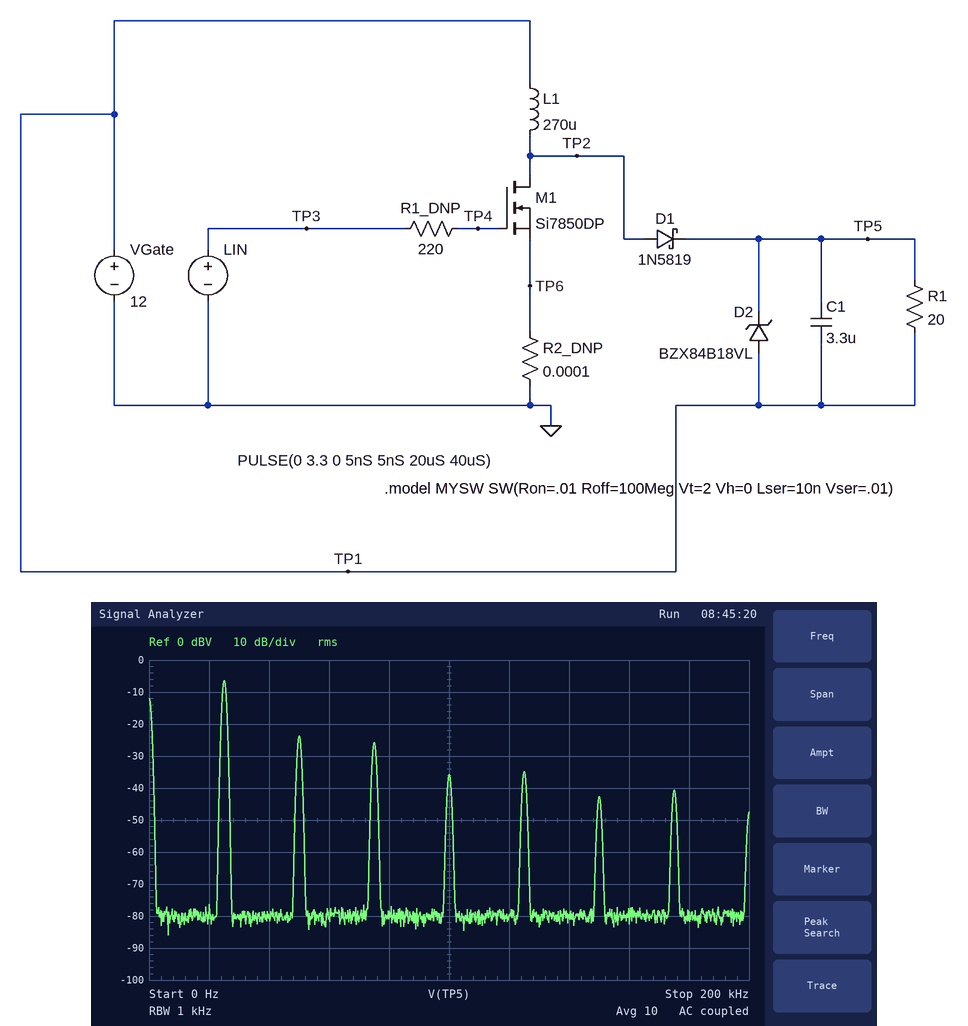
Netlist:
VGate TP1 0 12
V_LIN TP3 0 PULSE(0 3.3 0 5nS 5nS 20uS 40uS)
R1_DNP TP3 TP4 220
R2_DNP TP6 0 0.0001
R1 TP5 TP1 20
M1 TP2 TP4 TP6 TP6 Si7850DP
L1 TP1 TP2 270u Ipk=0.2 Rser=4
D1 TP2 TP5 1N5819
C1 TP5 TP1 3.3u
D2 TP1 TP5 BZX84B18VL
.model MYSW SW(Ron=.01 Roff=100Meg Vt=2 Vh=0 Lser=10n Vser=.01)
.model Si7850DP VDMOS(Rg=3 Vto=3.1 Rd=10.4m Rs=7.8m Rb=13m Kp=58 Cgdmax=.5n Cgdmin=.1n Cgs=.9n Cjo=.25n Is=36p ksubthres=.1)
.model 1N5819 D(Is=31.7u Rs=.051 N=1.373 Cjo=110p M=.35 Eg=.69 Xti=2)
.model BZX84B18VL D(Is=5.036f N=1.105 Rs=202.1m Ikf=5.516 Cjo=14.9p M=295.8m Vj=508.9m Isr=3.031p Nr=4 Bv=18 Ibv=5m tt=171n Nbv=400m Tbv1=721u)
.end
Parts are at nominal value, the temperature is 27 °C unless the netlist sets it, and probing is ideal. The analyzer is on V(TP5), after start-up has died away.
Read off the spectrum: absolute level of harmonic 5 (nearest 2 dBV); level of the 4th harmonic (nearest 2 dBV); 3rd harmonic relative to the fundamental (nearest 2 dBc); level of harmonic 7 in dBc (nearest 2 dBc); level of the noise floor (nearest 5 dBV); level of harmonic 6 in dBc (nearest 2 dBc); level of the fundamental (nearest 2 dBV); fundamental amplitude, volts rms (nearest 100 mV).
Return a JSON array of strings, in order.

["-34 dBV", "-36 dBV", "-20 dBc", "-34 dBc", "-80 dBV", "-36 dBc", "-6 dBV", "500 mV"]
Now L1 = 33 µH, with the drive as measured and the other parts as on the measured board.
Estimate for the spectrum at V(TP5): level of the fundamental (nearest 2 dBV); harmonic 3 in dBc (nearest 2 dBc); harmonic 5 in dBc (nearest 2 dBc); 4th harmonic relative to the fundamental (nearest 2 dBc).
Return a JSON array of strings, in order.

["-12 dBV", "-12 dBc", "-22 dBc", "-18 dBc"]
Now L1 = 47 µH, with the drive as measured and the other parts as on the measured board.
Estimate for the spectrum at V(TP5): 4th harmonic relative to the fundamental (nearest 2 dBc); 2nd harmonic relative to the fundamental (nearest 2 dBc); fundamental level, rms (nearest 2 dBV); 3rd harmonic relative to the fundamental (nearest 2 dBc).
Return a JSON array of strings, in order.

["-20 dBc", "-8 dBc", "-6 dBV", "-14 dBc"]
